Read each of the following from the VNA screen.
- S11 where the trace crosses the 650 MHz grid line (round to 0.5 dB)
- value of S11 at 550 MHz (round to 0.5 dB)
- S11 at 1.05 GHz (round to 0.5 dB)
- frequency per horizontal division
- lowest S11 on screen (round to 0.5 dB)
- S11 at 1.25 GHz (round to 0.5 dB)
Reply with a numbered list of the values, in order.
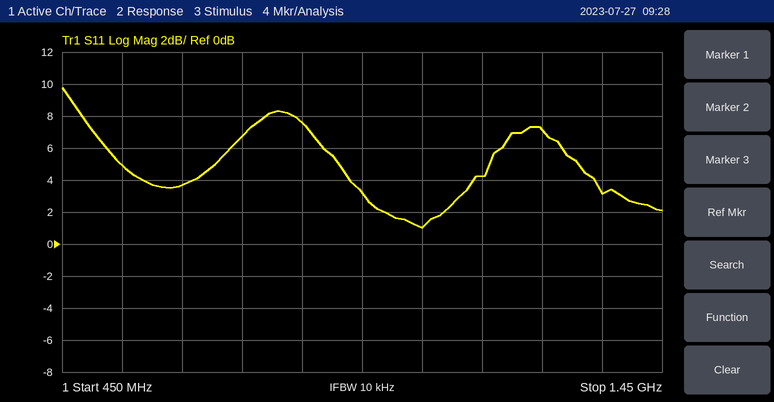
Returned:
1. 3.5 dB
2. 5.0 dB
3. 1.0 dB
4. 100 MHz
5. 1.0 dB
6. 7.0 dB
